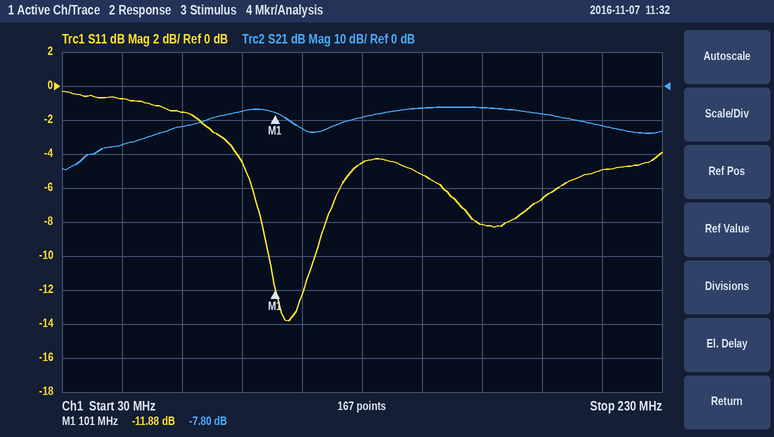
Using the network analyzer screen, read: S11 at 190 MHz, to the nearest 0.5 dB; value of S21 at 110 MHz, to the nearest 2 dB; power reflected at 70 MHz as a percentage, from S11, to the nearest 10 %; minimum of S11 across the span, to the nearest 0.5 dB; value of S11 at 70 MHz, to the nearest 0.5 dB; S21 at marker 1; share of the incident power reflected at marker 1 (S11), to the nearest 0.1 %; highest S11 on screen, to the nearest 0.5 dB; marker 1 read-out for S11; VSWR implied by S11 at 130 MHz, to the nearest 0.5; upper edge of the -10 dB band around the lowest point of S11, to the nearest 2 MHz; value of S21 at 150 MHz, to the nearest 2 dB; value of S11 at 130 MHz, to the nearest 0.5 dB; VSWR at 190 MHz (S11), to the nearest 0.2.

-6.5 dB
-12 dB
70 %
-14.0 dB
-1.5 dB
-7.80 dB
6.5 %
-0.5 dB
-11.88 dB
4.0
114 MHz
-6 dB
-4.5 dB
2.8
